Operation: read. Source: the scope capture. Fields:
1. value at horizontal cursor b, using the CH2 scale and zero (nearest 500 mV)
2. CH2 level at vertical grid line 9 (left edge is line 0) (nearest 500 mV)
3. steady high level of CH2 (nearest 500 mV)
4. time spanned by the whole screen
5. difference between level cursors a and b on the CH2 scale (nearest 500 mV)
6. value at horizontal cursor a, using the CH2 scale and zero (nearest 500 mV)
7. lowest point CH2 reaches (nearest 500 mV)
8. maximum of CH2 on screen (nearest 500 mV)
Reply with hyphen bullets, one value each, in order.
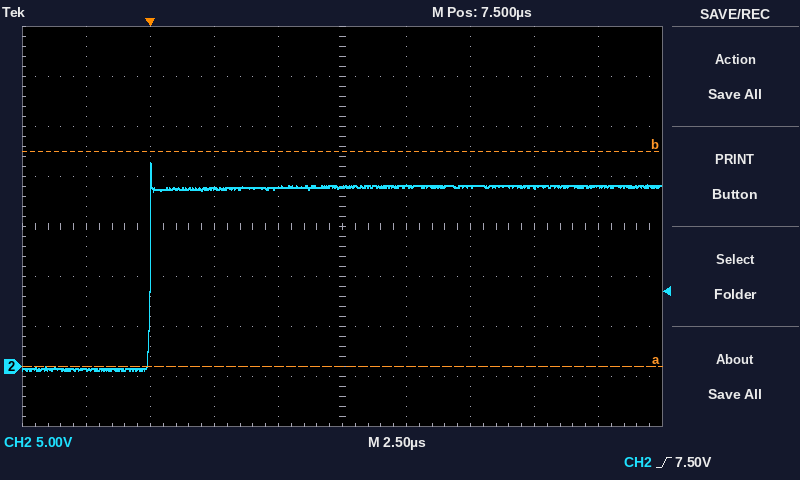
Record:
- 21.5 V
- 18.0 V
- 18.0 V
- 25 µs
- 21.5 V
- 0.0 V
- -500 mV
- 20.5 V
